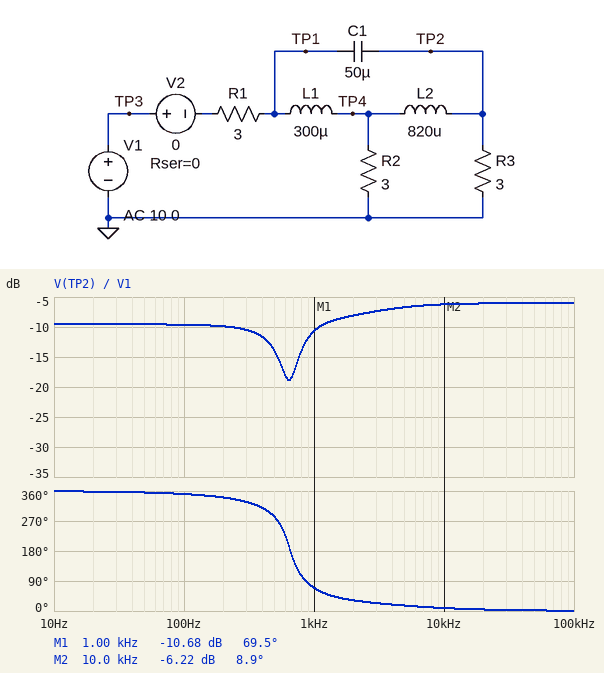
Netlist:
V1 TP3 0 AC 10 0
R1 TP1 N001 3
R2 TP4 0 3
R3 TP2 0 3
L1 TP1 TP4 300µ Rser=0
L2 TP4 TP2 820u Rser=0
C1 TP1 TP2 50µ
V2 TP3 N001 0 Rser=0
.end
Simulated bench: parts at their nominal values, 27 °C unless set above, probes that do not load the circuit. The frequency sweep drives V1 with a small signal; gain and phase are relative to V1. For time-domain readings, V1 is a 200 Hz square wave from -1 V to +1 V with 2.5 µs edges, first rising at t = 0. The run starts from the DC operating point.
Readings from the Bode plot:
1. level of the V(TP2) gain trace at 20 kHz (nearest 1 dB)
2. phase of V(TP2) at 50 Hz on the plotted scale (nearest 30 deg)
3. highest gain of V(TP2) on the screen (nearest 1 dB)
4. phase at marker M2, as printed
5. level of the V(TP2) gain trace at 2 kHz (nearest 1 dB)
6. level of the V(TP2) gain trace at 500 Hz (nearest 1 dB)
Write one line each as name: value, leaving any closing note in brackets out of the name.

level of the V(TP2) gain trace at 20 kHz: -6 dB
phase of V(TP2) at 50 Hz on the plotted scale: 360 deg
highest gain of V(TP2) on the screen: -6 dB
phase at marker M2, as printed: 8.9 deg
level of the V(TP2) gain trace at 2 kHz: -8 dB
level of the V(TP2) gain trace at 500 Hz: -14 dB
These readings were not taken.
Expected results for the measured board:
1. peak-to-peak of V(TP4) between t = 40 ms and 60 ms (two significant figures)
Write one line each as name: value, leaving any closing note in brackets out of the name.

peak-to-peak of V(TP4) between t = 40 ms and 60 ms: 910 mV
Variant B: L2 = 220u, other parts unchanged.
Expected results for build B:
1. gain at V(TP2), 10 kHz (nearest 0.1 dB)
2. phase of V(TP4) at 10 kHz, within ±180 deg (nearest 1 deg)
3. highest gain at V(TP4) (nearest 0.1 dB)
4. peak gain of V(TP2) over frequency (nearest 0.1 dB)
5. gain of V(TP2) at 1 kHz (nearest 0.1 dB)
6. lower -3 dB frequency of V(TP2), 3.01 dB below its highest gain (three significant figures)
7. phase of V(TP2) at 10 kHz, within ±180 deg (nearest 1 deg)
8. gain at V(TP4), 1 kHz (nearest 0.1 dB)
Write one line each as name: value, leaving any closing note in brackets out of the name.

gain at V(TP2), 10 kHz: -6.6 dB
phase of V(TP4) at 10 kHz, within ±180 deg: -60 deg
highest gain at V(TP4): -9.5 dB
peak gain of V(TP2) over frequency: -6.0 dB
gain of V(TP2) at 1 kHz: -15.7 dB
lower -3 dB frequency of V(TP2), 3.01 dB below its highest gain: 1.78 kHz
phase of V(TP2) at 10 kHz, within ±180 deg: 12 deg
gain at V(TP4), 1 kHz: -11.2 dB
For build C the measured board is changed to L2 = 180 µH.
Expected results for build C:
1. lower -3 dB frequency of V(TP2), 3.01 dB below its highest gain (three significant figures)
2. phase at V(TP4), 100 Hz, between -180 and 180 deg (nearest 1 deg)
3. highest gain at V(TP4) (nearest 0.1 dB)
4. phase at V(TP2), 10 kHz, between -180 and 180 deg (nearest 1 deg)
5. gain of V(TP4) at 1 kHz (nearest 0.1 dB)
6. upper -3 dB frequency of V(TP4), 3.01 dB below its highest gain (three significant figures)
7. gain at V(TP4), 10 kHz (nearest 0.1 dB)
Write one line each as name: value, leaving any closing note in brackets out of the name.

lower -3 dB frequency of V(TP2), 3.01 dB below its highest gain: 1.96 kHz
phase at V(TP4), 100 Hz, between -180 and 180 deg: -2 deg
highest gain at V(TP4): -9.5 dB
phase at V(TP2), 10 kHz, between -180 and 180 deg: 13 deg
gain of V(TP4) at 1 kHz: -12.3 dB
upper -3 dB frequency of V(TP4), 3.01 dB below its highest gain: 6.36 kHz
gain at V(TP4), 10 kHz: -14.9 dB
